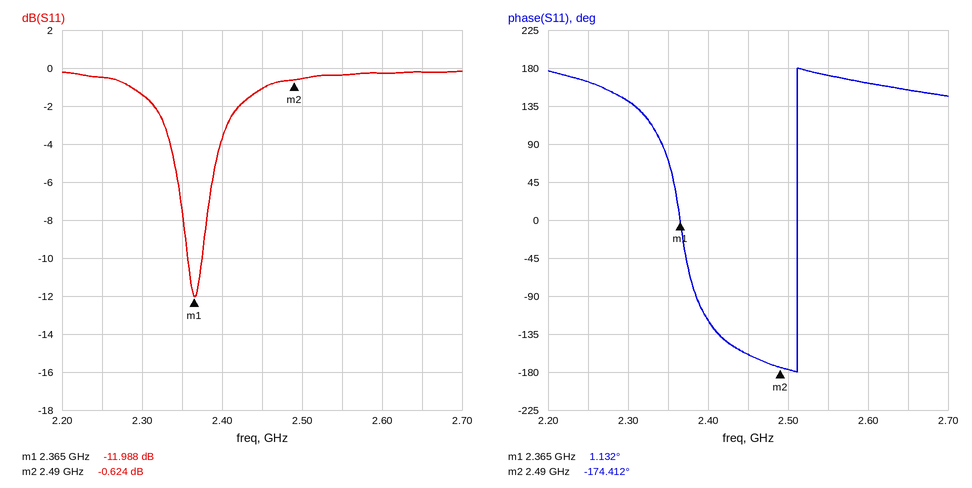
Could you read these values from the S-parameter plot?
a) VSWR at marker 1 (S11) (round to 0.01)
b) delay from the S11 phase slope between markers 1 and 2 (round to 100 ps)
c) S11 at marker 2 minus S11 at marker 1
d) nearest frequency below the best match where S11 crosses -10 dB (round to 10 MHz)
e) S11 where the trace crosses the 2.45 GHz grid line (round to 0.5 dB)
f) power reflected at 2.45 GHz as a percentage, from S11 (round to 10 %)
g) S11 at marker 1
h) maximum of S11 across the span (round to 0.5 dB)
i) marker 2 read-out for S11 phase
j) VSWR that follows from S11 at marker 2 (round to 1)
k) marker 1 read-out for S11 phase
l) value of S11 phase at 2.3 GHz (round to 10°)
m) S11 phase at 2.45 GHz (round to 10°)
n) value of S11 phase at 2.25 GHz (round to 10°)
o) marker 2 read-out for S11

1.67
3.9 ns
11.364 dB
2.36 GHz
-1.0 dB
80 %
-11.988 dB
0.0 dB
-174.412°
28
1.132°
140°
-160°
160°
-0.624 dB
